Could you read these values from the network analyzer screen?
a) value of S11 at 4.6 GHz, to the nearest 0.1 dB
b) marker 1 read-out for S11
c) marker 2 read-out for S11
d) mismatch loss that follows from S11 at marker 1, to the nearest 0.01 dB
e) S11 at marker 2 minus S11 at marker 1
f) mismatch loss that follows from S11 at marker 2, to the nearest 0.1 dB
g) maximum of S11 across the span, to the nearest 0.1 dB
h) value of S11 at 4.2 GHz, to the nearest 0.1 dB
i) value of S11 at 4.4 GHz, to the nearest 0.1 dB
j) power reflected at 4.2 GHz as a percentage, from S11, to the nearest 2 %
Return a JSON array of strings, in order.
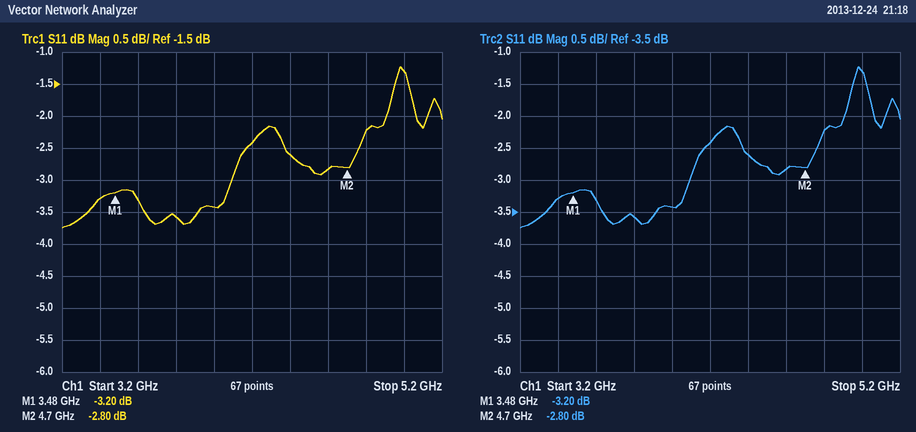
["-2.8 dB", "-3.20 dB", "-2.80 dB", "2.83 dB", "0.40 dB", "3.2 dB", "-1.2 dB", "-2.4 dB", "-2.6 dB", "58 %"]
